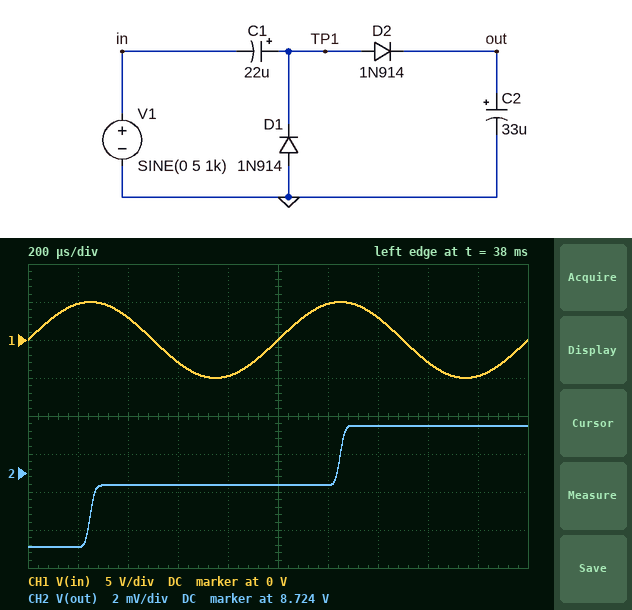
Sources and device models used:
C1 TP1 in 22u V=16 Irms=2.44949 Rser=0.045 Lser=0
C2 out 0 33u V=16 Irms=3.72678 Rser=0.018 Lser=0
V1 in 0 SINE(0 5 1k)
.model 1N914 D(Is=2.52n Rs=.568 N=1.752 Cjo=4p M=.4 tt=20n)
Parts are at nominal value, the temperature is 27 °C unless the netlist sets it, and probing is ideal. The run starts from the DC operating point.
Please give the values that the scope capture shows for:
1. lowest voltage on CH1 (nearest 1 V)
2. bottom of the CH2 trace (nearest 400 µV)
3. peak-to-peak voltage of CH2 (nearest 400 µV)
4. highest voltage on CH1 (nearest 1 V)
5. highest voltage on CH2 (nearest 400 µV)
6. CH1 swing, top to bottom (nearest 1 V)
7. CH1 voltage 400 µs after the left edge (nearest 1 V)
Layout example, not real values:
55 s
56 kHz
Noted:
-5 V
8.7200 V
6.4 mV
5 V
8.7264 V
10 V
3 V
